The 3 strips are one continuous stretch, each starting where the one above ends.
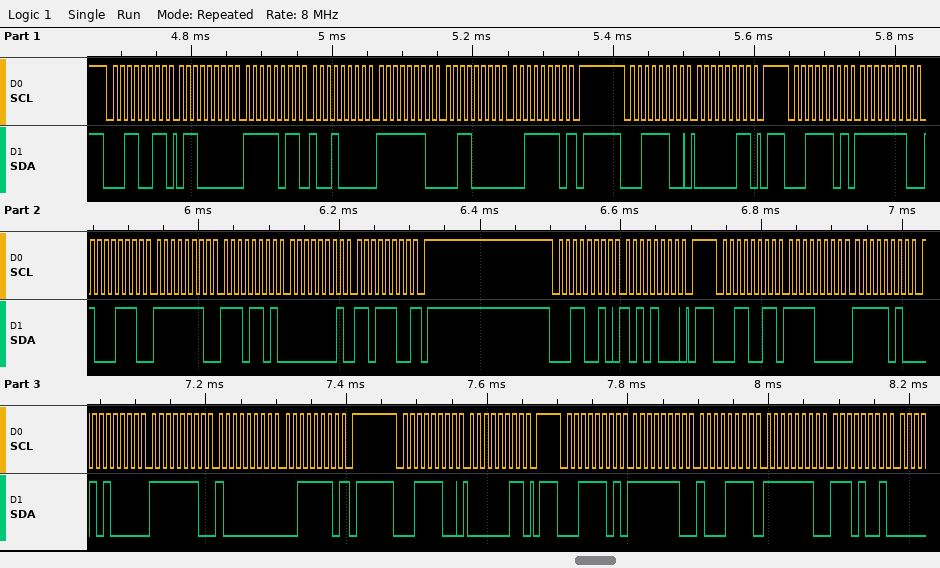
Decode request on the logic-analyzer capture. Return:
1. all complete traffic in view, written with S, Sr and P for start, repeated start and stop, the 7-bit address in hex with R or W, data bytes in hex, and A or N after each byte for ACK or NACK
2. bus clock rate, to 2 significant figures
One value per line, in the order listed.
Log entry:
S 19R A 60 A FB A 90 A FE A 30 A 3E N P S 1EW A 03 A P S 1ER A FE A 8E A FE A ED A 01 A DC N P S 19W A A8 A P S 19R A F0 A FA A 50 A FE A 80 A 3E N P S 1EW A 03 A P S 1ER A FE A 8F A FE A E9 A
100 kHz
